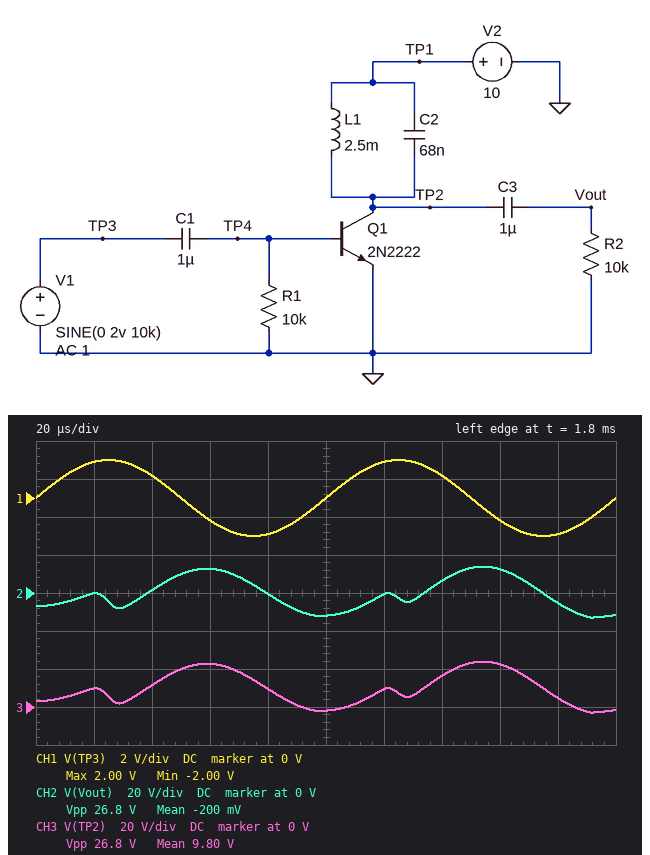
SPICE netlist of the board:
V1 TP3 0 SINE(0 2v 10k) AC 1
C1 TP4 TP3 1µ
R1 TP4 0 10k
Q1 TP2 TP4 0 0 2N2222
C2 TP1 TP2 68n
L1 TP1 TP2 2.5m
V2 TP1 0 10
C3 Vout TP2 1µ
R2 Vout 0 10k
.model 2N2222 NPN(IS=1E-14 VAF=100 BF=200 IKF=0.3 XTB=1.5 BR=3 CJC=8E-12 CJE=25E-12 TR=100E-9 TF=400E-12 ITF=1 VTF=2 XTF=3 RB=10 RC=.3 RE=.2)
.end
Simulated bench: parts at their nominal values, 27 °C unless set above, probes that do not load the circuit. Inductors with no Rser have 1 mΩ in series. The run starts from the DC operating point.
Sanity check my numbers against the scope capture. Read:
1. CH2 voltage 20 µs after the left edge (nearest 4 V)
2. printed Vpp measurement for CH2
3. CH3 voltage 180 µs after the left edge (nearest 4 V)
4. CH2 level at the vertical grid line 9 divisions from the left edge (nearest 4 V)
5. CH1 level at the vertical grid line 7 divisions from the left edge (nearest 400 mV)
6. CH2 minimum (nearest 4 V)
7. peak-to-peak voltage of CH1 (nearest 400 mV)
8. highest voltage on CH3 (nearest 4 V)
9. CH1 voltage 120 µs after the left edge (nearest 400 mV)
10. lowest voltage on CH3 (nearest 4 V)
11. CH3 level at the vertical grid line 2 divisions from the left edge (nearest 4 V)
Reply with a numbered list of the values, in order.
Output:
1. 0 V
2. 26.8 V
3. 4 V
4. -4 V
5. 1.2 V
6. -12 V
7. 4.0 V
8. 24 V
9. 2.0 V
10. -4 V
11. 12 V
